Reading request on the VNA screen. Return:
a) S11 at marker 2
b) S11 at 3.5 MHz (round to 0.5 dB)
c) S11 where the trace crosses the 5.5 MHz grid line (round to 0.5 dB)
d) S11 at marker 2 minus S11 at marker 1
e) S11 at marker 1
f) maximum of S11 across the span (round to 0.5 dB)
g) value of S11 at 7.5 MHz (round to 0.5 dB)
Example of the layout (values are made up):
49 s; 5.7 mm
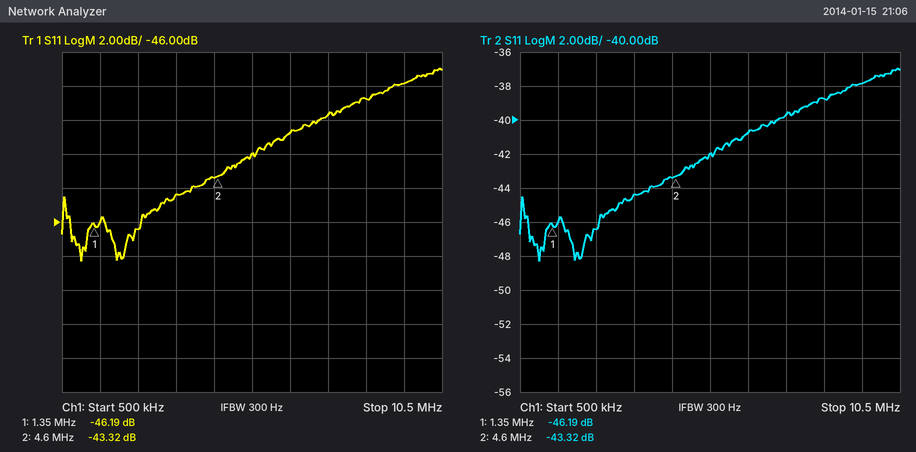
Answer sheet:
-43.32 dB; -44.5 dB; -42.0 dB; 2.87 dB; -46.19 dB; -37.0 dB; -39.5 dB
